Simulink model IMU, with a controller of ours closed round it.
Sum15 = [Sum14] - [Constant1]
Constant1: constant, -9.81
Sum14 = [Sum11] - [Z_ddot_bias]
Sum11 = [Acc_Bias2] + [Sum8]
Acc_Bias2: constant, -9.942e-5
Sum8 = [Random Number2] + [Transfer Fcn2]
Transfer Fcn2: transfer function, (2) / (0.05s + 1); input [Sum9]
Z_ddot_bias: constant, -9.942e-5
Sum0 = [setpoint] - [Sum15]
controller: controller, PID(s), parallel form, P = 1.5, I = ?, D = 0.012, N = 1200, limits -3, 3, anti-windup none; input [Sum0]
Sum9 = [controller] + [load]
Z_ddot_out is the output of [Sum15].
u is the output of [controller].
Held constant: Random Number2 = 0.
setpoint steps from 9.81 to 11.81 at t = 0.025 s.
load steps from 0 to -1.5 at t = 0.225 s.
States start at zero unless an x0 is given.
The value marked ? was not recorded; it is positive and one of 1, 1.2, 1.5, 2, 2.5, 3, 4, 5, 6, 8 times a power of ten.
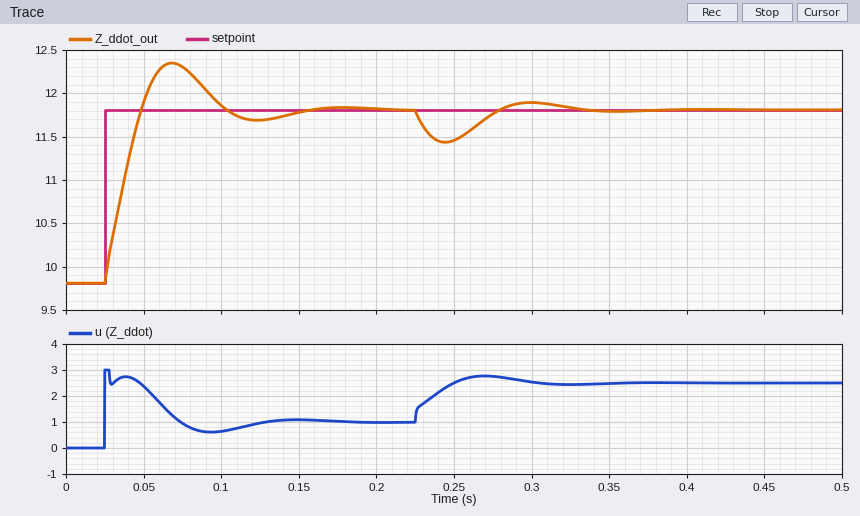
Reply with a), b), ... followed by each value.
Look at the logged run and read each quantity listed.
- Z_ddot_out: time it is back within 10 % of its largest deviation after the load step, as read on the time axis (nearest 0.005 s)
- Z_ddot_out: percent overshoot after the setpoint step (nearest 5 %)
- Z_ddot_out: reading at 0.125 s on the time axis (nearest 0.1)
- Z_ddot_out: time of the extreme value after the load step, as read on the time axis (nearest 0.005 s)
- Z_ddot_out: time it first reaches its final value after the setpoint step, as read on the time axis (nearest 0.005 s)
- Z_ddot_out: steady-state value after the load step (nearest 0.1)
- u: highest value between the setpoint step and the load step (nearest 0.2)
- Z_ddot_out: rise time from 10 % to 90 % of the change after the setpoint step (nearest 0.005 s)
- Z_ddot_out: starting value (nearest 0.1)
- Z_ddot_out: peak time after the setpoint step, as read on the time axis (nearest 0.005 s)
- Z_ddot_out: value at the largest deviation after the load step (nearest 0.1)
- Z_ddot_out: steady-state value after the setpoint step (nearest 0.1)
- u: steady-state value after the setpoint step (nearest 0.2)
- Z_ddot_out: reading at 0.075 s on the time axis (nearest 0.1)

a) 0.320 s
b) 25 %
c) 11.7
d) 0.245 s
e) 0.050 s
f) 11.8
g) 3.0
h) 0.020 s
i) 9.8
j) 0.070 s
k) 11.4
l) 11.8
m) 1.0
n) 12.3
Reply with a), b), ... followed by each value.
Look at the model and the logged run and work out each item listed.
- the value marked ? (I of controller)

a) 150
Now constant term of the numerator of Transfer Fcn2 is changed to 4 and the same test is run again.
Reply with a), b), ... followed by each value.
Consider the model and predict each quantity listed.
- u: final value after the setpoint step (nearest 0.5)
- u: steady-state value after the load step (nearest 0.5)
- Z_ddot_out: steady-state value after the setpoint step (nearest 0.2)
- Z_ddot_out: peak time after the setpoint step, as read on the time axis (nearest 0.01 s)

a) 0.5
b) 2.0
c) 11.8
d) 0.06 s
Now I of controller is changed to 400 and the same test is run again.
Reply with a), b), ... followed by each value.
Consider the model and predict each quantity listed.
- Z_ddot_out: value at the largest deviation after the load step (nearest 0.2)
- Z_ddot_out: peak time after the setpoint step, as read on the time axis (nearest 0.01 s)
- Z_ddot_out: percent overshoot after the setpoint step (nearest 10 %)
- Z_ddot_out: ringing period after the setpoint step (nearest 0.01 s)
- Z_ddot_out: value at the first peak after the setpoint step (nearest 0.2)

a) 11.6
b) 0.06 s
c) 50 %
d) 0.06 s
e) 12.8
